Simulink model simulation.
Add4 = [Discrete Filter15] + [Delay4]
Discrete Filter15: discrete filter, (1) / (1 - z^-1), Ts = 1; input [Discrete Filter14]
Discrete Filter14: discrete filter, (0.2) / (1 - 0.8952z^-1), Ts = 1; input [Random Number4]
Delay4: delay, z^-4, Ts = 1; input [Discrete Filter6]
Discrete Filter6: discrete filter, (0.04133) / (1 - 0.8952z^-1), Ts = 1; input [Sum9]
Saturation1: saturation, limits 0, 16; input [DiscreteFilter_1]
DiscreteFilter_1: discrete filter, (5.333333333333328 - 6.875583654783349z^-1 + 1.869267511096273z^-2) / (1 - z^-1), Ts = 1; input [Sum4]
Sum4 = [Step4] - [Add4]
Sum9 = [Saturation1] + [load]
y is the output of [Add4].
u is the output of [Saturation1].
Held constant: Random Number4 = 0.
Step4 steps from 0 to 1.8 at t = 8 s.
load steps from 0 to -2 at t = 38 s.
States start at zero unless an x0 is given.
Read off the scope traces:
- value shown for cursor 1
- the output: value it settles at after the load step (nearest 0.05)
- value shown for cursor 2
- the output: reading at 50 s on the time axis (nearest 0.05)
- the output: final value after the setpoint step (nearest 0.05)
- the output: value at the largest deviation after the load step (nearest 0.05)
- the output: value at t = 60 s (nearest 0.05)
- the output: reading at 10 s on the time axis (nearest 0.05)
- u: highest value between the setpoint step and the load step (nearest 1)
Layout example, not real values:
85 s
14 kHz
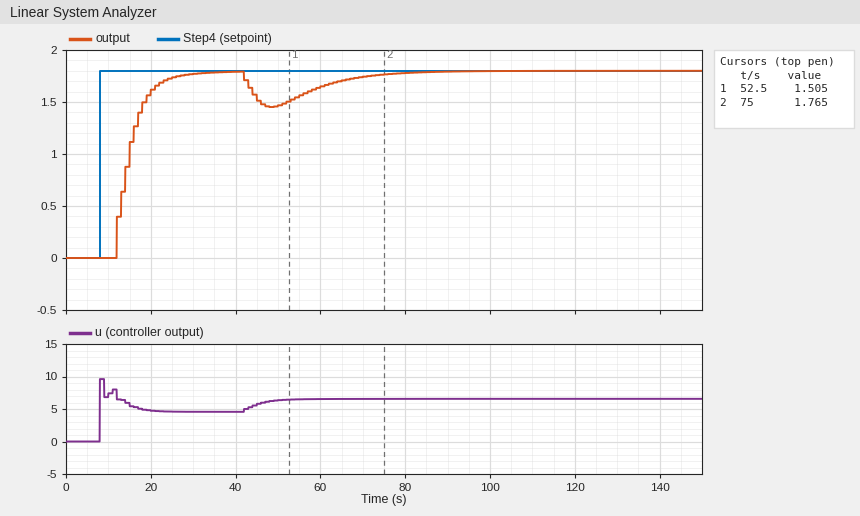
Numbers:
1.505
1.80
1.765
1.45
1.80
1.45
1.65
0.00
10
